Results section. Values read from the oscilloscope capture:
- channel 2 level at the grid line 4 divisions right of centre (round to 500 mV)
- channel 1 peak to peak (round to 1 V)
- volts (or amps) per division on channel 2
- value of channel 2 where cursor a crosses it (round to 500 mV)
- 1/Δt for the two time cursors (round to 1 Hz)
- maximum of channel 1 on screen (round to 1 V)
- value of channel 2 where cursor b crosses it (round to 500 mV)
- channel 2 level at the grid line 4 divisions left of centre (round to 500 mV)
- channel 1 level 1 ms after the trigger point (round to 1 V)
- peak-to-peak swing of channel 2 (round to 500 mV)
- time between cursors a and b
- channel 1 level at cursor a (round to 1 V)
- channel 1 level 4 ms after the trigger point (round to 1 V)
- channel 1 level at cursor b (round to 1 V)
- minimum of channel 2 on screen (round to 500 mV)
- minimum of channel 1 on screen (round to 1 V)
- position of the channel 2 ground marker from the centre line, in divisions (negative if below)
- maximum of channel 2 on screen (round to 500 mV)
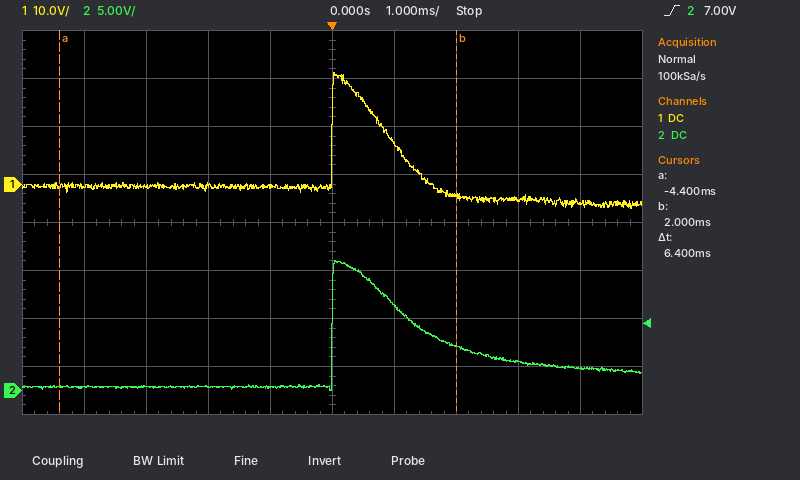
2.5 V
28 V
5 V
500 mV
156 Hz
23 V
4.5 V
500 mV
9 V
13.5 V
6.4 ms
0 V
-4 V
-3 V
0.0 V
-5 V
-3.5 div
13.5 V
